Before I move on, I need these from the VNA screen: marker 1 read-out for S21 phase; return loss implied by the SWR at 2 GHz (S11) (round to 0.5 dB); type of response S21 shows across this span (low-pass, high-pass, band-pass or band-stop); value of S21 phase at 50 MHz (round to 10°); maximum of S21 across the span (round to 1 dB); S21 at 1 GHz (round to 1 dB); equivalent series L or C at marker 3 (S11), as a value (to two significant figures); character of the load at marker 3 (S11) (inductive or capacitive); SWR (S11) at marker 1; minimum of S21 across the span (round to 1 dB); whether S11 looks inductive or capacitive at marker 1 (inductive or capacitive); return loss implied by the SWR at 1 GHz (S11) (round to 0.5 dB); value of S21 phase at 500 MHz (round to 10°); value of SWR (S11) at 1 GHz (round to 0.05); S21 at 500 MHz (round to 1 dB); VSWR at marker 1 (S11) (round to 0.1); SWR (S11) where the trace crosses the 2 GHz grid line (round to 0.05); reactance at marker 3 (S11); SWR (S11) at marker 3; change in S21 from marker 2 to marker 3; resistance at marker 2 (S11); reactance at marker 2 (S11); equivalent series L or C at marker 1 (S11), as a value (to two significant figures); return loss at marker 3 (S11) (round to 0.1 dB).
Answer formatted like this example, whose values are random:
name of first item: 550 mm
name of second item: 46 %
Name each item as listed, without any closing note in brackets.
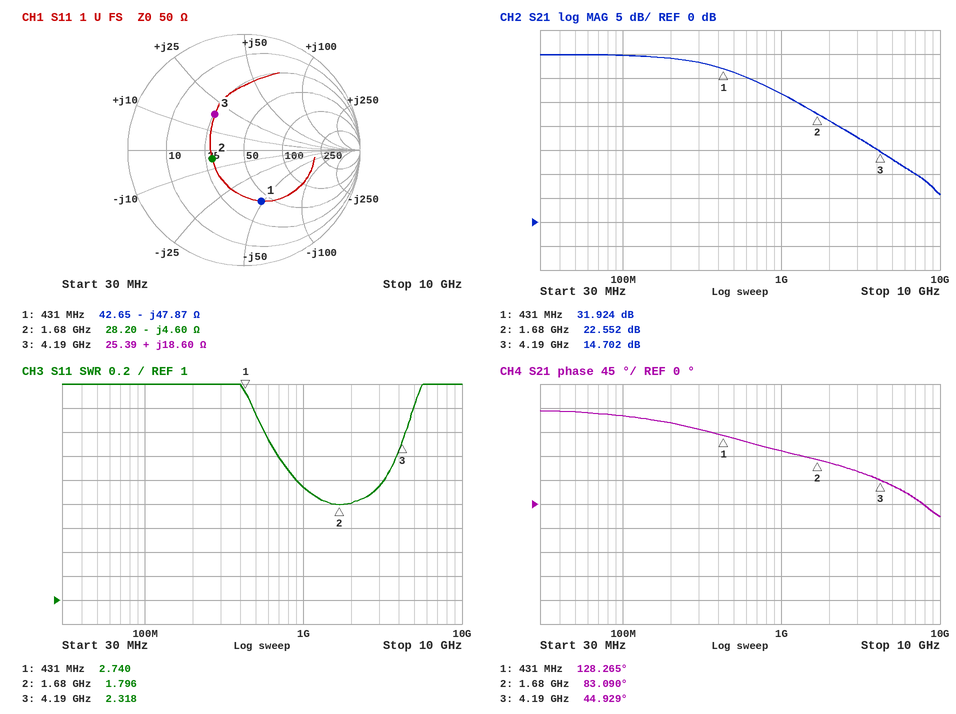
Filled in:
marker 1 read-out for S21 phase: 128.265°
return loss implied by the SWR at 2 GHz (S11): 11.0 dB
type of response S21 shows across this span: low-pass
value of S21 phase at 50 MHz: 170°
maximum of S21 across the span: 35 dB
S21 at 1 GHz: 27 dB
equivalent series L or C at marker 3 (S11), as a value: 710 pH
character of the load at marker 3 (S11): inductive
SWR (S11) at marker 1: 2.740
minimum of S21 across the span: 6 dB
whether S11 looks inductive or capacitive at marker 1: capacitive
return loss implied by the SWR at 1 GHz (S11): 10.0 dB
value of S21 phase at 500 MHz: 120°
value of SWR (S11) at 1 GHz: 1.95
S21 at 500 MHz: 31 dB
VSWR at marker 1 (S11): 2.7
SWR (S11) where the trace crosses the 2 GHz grid line: 1.80
reactance at marker 3: +18.60 Ω
SWR (S11) at marker 3: 2.318
change in S21 from marker 2 to marker 3: -7.850 dB
resistance at marker 2: 28.20 Ω
reactance at marker 2: -4.60 Ω
equivalent series L or C at marker 1 (S11), as a value: 7.7 pF
return loss at marker 3 (S11): 8.0 dB
